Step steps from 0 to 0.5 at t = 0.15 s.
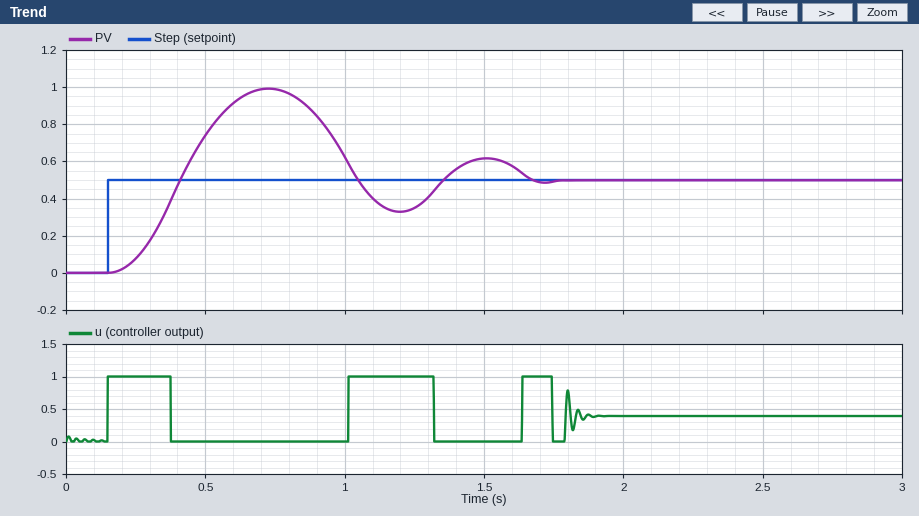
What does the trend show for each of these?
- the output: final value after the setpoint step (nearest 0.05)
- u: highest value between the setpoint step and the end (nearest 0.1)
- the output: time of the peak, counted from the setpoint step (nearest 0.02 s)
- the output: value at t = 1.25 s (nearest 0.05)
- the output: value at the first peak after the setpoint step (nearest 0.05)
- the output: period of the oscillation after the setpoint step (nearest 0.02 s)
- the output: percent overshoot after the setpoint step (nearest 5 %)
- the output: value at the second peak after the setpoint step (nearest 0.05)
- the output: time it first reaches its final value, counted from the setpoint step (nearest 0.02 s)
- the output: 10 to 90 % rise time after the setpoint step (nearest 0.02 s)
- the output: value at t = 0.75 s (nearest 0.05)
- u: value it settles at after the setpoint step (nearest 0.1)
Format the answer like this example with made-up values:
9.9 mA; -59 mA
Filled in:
0.50; 1.0; 0.58 s; 0.35; 1.00; 0.78 s; 100 %; 0.60; 0.26 s; 0.16 s; 1.00; 0.4
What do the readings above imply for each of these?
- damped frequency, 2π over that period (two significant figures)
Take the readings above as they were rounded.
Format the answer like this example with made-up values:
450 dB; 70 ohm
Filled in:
8.1 rad/s
